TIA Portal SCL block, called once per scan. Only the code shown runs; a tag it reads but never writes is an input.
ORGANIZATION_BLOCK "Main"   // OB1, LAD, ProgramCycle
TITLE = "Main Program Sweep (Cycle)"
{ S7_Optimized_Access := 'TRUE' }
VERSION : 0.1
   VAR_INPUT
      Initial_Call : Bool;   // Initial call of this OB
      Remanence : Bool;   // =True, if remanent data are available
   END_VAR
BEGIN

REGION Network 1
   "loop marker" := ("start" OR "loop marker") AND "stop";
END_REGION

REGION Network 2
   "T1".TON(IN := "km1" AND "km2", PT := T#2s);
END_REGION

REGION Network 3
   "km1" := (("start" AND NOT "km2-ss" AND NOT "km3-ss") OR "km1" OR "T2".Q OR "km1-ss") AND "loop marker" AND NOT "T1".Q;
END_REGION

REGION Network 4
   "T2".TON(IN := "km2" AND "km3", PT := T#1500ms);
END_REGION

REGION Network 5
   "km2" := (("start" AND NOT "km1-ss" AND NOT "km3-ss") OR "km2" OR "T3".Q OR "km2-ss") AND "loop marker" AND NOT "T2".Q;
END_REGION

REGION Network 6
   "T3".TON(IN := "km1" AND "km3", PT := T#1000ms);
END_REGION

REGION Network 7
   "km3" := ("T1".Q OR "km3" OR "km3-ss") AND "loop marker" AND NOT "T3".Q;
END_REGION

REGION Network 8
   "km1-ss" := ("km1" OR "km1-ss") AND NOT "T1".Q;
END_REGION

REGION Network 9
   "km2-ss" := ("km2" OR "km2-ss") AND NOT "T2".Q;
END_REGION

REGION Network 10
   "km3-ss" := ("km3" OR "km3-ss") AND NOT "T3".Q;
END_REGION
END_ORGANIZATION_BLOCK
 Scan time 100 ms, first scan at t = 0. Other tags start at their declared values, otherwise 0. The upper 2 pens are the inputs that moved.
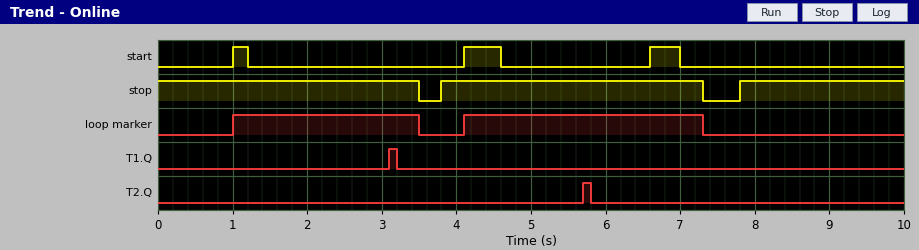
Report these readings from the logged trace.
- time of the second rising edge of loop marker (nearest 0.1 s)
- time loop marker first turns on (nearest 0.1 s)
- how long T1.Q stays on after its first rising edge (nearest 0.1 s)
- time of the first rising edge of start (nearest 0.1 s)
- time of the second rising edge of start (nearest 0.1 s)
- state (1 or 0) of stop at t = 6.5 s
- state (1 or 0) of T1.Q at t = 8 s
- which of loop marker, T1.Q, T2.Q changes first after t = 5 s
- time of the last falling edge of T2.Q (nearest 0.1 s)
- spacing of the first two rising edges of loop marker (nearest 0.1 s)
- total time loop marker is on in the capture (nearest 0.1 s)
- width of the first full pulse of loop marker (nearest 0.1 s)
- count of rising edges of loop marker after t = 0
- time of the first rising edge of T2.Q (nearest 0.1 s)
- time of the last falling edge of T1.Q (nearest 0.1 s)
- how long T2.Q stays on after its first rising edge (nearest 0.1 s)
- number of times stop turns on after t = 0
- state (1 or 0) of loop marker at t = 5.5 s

4.1 s
1.0 s
0.1 s
1.0 s
4.1 s
1
0
T2.Q
5.8 s
3.1 s
5.7 s
2.5 s
2
5.7 s
3.2 s
0.1 s
2
1
